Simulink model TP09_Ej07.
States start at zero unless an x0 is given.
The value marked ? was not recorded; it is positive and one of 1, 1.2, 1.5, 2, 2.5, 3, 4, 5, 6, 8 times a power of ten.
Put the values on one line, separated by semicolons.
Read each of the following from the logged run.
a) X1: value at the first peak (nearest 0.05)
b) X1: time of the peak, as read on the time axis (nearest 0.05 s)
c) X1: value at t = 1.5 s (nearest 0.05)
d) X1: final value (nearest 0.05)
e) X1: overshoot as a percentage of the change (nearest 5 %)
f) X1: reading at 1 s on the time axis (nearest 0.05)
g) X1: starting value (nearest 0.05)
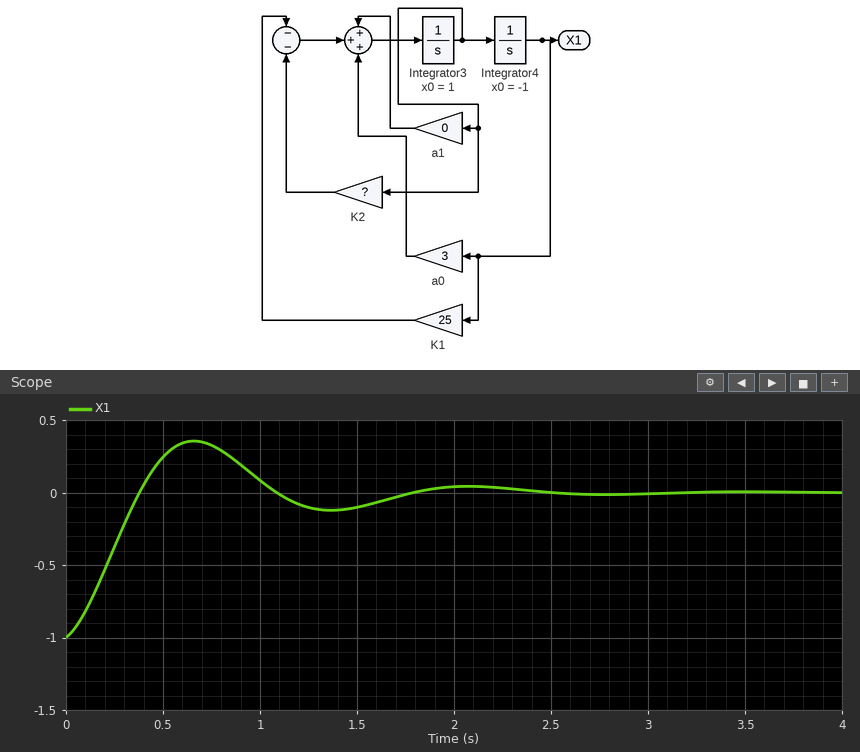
0.35; 0.65 s; -0.10; 0.00; 35 %; 0.10; -1.00
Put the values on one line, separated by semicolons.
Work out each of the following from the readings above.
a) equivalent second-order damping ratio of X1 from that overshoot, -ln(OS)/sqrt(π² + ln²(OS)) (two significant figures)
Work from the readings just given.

0.32
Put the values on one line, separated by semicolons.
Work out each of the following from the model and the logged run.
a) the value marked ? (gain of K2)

3
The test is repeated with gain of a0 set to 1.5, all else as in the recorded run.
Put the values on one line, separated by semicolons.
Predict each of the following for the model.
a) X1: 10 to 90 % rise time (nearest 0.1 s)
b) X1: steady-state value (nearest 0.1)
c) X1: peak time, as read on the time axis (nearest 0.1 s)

0.3 s; 0.0; 0.6 s
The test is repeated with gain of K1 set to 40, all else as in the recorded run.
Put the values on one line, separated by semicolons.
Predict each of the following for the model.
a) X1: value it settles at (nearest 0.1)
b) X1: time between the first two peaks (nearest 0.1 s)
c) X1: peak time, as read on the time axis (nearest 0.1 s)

0.0; 1.1 s; 0.5 s
